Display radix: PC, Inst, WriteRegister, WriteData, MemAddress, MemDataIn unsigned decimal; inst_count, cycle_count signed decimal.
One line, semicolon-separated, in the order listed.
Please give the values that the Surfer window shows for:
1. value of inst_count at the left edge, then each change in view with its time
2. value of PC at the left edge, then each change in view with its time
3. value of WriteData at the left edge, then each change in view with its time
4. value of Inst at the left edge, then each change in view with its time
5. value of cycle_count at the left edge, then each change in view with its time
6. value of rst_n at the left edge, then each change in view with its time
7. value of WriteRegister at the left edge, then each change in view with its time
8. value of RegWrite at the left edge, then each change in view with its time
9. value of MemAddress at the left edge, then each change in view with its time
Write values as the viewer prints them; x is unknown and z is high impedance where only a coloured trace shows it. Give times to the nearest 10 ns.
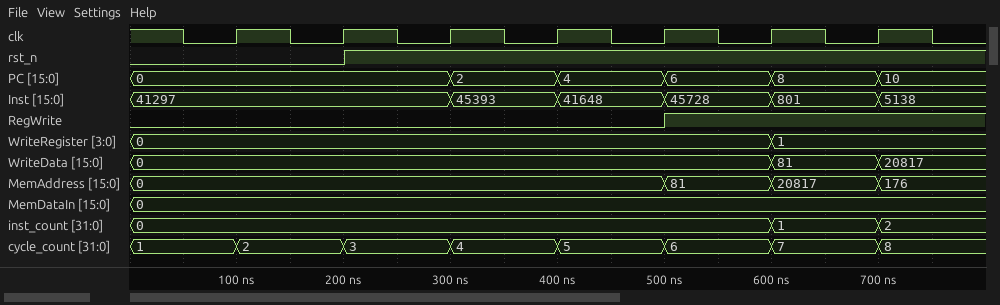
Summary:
0, 1 at 600 ns, 2 at 700 ns; 0, 2 at 300 ns, 4 at 400 ns, 6 at 500 ns, 8 at 600 ns, 10 at 700 ns; 0, 81 at 600 ns, 20817 at 700 ns; 41297, 45393 at 300 ns, 41648 at 400 ns, 45728 at 500 ns, 801 at 600 ns, 5138 at 700 ns; 1, 2 at 100 ns, 3 at 200 ns, 4 at 300 ns, 5 at 400 ns, 6 at 500 ns, 7 at 600 ns, 8 at 700 ns; 0, 1 at 200 ns; 0, 1 at 600 ns; 0, 1 at 500 ns; 0, 81 at 500 ns, 20817 at 600 ns, 176 at 700 ns
